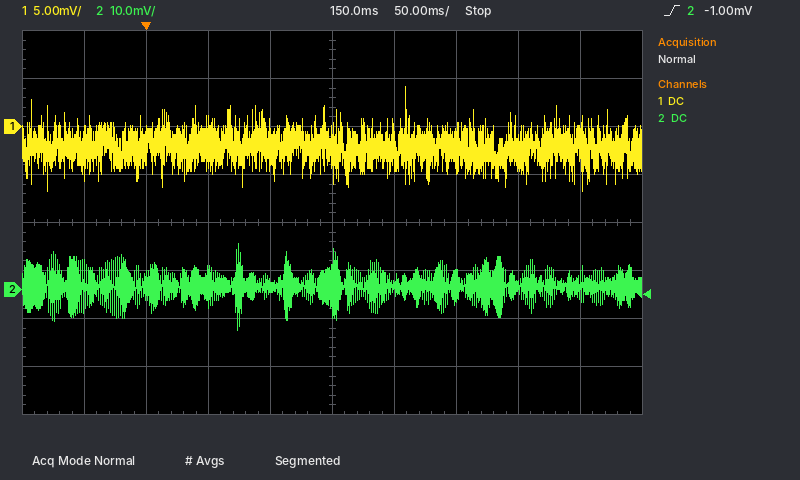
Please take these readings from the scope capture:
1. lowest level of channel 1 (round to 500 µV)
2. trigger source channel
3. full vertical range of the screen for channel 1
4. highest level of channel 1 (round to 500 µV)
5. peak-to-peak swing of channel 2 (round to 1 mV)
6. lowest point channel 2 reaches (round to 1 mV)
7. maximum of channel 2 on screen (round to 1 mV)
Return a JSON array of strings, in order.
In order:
["-6.5 mV", "channel 2", "40 mV", "4.0 mV", "18 mV", "-8 mV", "10 mV"]
